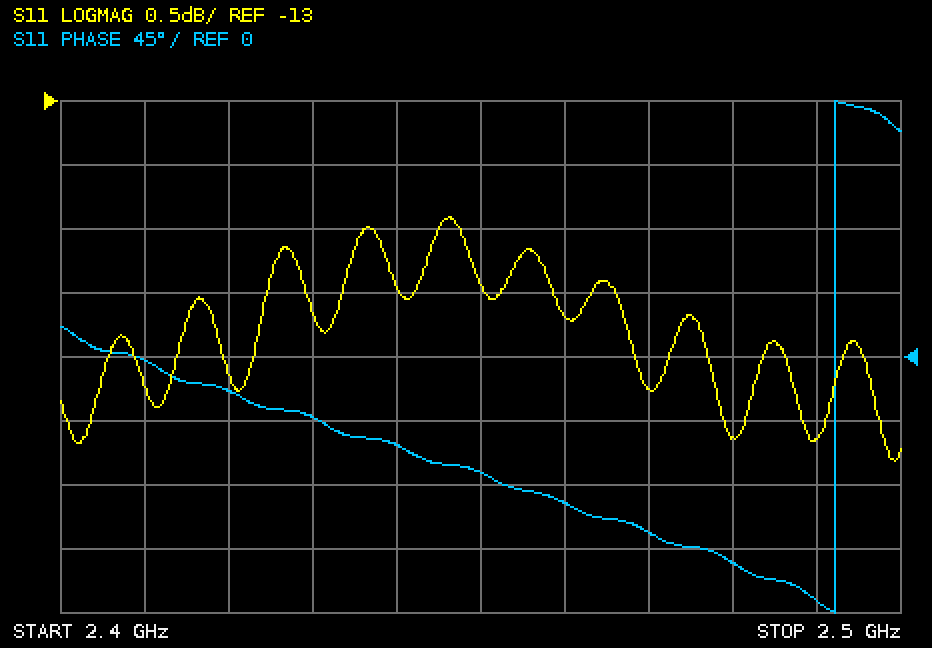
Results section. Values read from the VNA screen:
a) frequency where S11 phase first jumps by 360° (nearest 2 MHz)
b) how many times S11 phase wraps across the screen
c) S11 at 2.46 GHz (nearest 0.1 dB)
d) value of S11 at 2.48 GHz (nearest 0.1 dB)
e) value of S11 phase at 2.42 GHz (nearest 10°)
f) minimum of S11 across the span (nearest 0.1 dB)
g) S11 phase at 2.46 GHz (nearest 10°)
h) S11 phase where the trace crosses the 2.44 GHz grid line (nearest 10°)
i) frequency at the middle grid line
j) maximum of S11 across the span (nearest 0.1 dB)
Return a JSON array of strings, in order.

["2.492 GHz", "1", "-14.7 dB", "-15.6 dB", "-20°", "-15.8 dB", "-100°", "-60°", "2.45 GHz", "-13.9 dB"]
